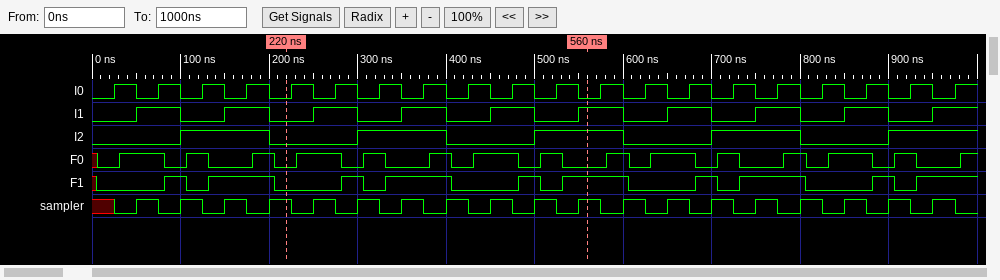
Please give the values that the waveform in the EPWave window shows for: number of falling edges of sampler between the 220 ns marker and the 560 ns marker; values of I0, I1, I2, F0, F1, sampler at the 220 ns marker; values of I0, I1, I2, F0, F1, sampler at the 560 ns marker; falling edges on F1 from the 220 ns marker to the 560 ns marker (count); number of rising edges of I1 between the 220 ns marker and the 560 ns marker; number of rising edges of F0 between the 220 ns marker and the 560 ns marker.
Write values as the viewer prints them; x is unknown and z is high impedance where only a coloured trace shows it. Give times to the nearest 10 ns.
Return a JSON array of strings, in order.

["7", "I0=0, I1=0, I2=0, F0=0, F1=0, sampler=1", "I0=0, I1=1, I2=1, F0=0, F1=1, sampler=1", "3", "4", "5"]
